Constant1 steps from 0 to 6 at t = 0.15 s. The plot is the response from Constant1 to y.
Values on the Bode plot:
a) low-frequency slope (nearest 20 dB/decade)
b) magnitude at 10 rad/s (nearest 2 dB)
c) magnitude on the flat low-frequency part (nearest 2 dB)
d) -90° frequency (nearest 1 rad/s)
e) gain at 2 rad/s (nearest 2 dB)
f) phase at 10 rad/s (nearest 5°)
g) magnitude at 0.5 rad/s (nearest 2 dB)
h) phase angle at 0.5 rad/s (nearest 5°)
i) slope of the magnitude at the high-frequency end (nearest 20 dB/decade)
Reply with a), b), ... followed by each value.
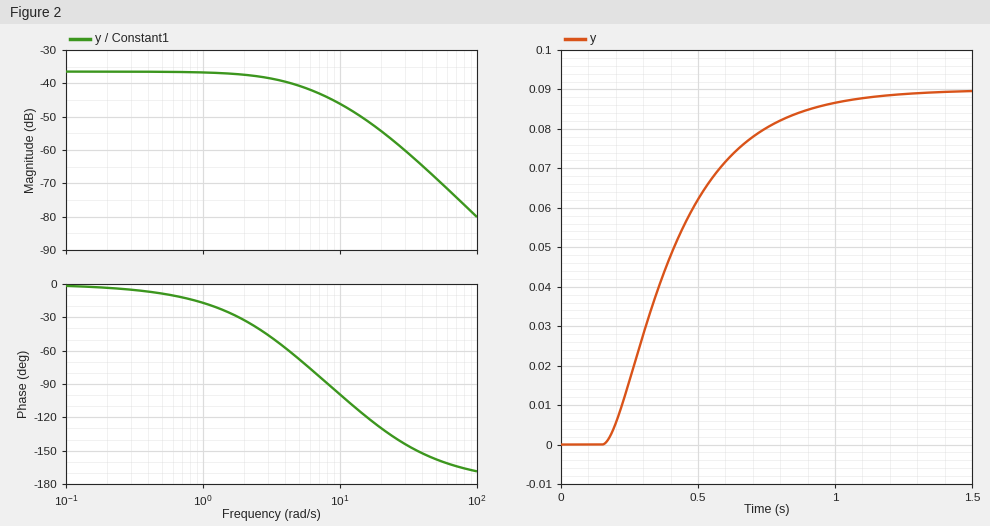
a) 0 dB/decade
b) -46 dB
c) -36 dB
d) 8 rad/s
e) -38 dB
f) -100°
g) -36 dB
h) -10°
i) -40 dB/decade
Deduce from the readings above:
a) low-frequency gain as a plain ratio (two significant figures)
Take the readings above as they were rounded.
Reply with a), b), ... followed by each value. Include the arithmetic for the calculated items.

a) 10^(-36 / 20) = 0.016
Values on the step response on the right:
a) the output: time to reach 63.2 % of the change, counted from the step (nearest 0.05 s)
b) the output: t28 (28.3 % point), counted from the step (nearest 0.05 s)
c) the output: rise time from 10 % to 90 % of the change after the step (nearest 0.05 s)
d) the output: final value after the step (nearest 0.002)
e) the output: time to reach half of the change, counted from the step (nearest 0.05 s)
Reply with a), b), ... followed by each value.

a) 0.30 s
b) 0.15 s
c) 0.55 s
d) 0.090
e) 0.25 s
